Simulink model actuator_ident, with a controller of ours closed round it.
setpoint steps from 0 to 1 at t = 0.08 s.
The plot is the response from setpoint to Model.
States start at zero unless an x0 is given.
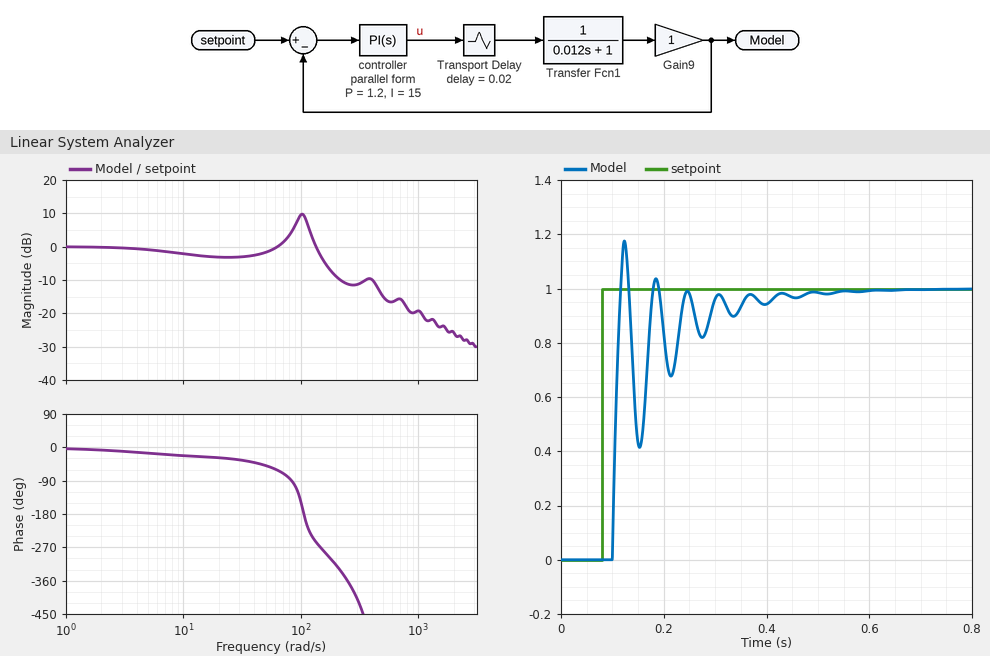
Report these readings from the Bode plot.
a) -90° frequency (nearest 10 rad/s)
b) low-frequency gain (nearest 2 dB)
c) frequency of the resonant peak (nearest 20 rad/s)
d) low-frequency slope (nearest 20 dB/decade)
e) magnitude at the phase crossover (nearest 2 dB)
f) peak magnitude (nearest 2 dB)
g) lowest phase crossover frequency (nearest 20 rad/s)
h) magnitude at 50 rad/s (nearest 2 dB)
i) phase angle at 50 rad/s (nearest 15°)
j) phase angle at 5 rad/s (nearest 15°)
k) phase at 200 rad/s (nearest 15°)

80 rad/s
0 dB
100 rad/s
0 dB/decade
10 dB
10 dB
100 rad/s
-2 dB
-45°
-15°
-315°
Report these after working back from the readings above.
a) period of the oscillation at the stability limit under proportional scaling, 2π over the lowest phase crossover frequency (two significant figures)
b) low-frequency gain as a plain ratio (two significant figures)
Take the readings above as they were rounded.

0.063 s
1.0
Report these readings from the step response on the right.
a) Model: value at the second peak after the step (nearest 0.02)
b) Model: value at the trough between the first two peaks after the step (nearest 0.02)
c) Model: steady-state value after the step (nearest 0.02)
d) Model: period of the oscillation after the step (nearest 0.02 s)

1.04
0.42
1.00
0.06 s
